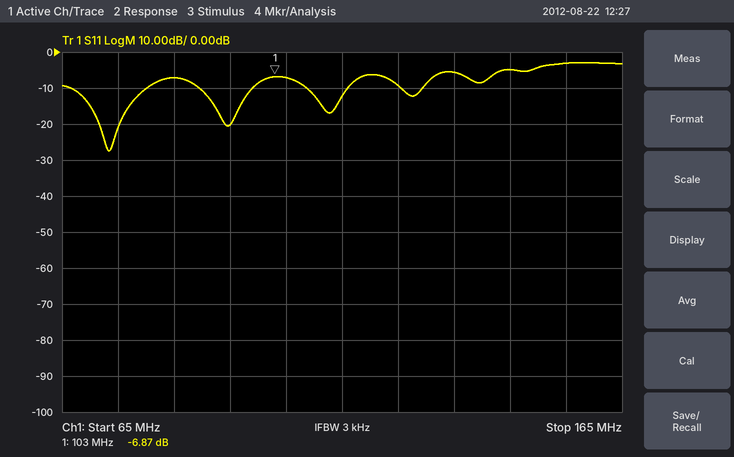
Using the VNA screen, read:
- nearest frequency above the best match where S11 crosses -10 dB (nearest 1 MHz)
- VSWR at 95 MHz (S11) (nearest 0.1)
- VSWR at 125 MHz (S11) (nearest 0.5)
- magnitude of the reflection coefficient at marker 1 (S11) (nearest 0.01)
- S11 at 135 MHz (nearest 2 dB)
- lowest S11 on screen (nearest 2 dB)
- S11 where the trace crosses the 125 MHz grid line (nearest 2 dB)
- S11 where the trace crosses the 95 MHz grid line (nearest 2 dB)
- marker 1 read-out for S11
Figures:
80 MHz
1.2
2.0
0.45
-6 dB
-28 dB
-10 dB
-20 dB
-6.87 dB
